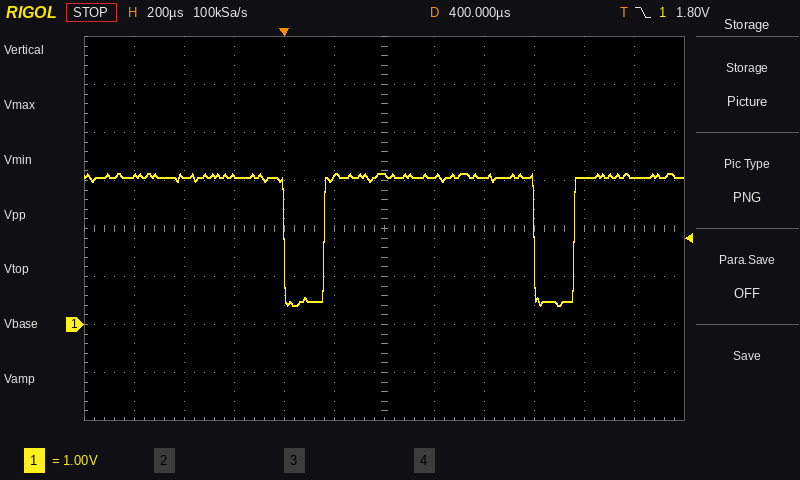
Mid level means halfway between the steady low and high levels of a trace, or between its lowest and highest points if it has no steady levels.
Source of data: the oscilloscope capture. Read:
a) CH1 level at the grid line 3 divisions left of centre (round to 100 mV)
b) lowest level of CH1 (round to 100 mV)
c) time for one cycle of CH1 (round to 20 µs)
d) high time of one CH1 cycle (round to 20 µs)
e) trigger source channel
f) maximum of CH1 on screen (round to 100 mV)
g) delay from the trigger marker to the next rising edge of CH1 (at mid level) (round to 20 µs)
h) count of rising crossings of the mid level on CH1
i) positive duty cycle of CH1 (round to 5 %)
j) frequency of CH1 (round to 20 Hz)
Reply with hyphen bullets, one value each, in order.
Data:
- 3.1 V
- 400 mV
- 1.00 ms
- 840 µs
- CH1
- 3.1 V
- 160 µs
- 2
- 85 %
- 1.00 kHz
